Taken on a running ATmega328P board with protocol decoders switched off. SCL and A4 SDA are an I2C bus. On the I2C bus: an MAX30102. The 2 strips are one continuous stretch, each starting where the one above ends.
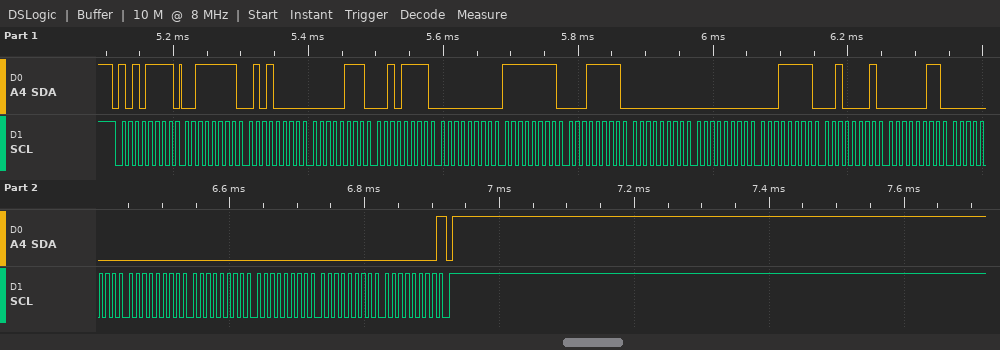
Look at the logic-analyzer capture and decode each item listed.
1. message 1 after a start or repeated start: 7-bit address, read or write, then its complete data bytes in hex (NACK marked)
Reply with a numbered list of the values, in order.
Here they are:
1. 0x57 read: 3F 50 07 2F 00 FF 1F 00 00 1F 21 03 00 00 00 00 00 00 NACK
